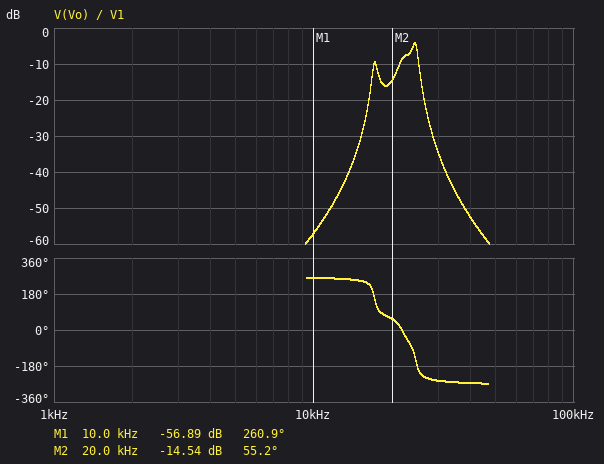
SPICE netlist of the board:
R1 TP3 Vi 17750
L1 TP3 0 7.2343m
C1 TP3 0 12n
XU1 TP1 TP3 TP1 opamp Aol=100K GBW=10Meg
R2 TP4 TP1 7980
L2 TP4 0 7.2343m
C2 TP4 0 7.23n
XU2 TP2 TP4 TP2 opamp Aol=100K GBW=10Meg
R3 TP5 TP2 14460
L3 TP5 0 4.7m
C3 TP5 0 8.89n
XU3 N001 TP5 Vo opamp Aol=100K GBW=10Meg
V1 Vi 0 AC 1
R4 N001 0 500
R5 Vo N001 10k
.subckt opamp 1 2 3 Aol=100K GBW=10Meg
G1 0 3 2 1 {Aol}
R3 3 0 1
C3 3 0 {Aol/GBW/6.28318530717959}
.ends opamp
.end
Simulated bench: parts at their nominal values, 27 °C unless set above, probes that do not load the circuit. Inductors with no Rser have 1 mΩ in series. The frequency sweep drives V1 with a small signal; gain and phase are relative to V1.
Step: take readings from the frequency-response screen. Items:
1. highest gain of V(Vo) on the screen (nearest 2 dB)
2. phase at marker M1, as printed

-4 dB
260.9 deg
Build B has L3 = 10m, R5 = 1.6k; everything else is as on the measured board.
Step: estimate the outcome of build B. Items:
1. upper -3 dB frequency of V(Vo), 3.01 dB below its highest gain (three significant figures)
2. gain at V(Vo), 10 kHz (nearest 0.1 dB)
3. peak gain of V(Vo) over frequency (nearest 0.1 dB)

17.4 kHz
-62.1 dB
-0.4 dB
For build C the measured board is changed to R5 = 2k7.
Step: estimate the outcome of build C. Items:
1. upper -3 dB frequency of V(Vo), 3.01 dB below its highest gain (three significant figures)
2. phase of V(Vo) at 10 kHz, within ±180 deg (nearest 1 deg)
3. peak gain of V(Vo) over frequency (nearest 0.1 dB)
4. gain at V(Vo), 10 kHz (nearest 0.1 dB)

25.0 kHz
-98 deg
-14.5 dB
-67.2 dB
